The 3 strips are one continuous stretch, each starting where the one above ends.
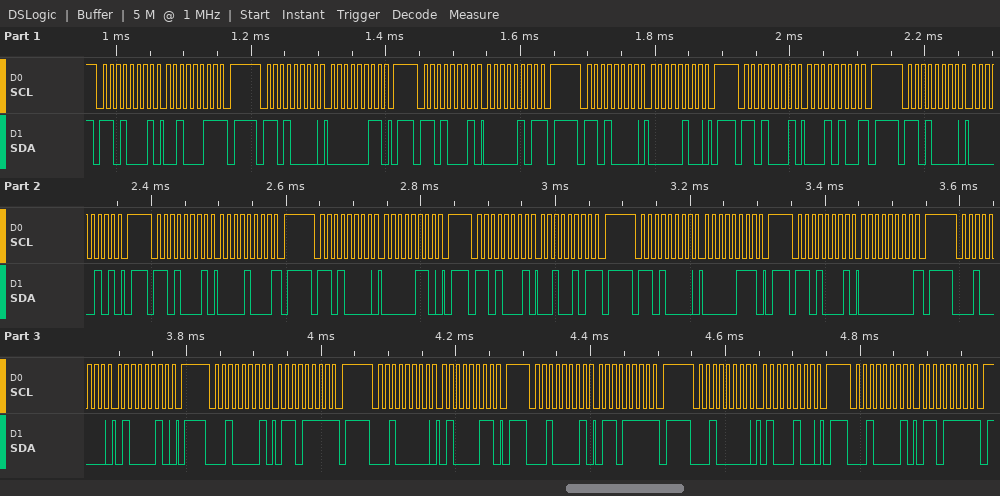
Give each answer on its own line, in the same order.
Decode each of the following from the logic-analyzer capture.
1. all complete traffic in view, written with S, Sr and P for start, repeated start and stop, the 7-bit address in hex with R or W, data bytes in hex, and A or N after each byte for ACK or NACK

S 68R A 23 N P S 68W A 03 A P S 68R A 05 N P S 68W A 04 A P S 68R A 14 N P S 68W A 05 A P S 68R A 08 N P S 68W A 06 A P S 68R A 25 N P S 68W A 07 A P S 68R A 00 N P S 10W A 42 A P S 10R A 6F N P S 10W A 43 A P S 10R A 6F N P S 10W A 44 A P S 10R A 6F N P
